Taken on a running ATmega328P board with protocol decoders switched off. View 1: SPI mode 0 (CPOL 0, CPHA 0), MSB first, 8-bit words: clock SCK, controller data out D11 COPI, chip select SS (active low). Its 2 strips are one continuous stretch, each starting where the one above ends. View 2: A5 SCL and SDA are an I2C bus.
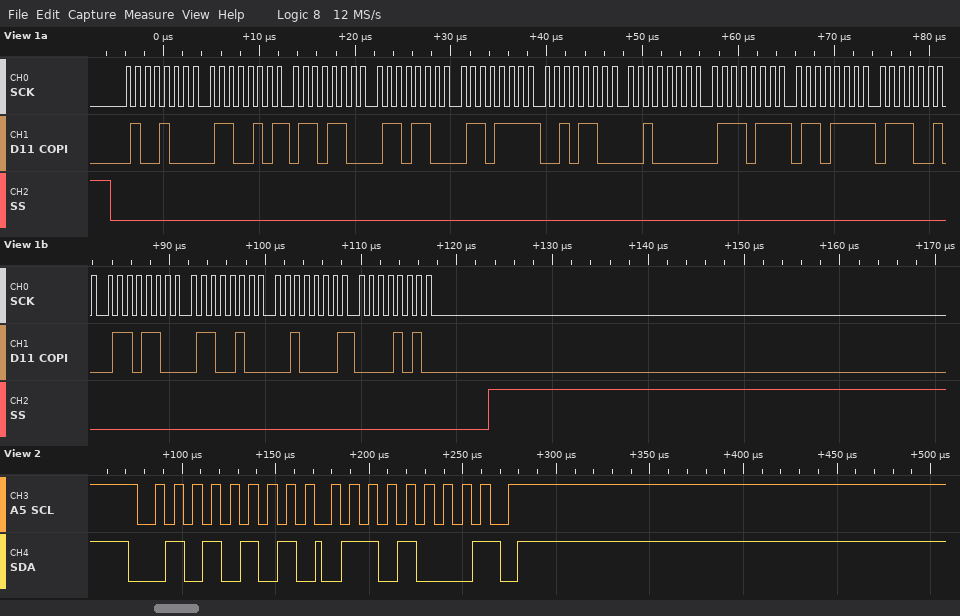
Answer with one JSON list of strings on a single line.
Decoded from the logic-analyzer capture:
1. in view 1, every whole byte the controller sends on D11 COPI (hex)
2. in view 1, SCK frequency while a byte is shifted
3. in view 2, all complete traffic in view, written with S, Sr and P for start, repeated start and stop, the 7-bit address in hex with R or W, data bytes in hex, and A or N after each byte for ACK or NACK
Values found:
["0x48 0x65 0x6C 0x6C 0x6F 0x2C 0x20 0x77 0x6F 0x72 0x6C 0x64 0x21 0x0A", "1 MHz", "S 2AR A 68 N P"]
